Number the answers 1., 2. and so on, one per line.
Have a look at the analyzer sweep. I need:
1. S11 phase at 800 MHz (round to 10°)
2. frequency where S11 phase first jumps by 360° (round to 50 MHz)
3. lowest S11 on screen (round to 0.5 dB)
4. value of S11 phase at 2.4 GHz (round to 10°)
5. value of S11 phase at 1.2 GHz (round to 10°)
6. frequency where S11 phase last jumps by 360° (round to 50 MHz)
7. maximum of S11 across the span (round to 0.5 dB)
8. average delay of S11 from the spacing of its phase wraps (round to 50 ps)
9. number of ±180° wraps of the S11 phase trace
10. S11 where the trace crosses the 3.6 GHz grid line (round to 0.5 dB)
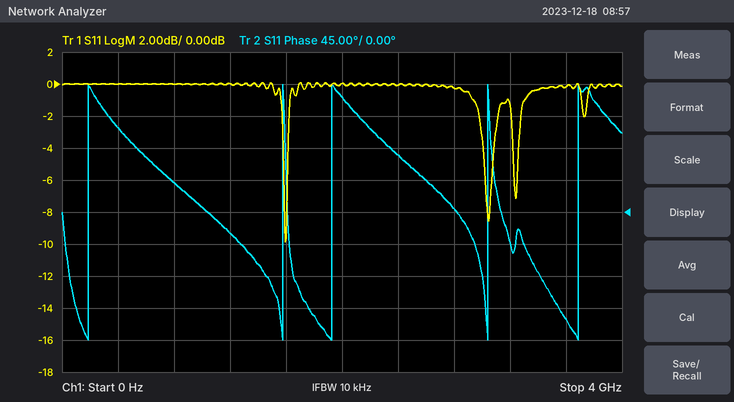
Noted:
1. 40°
2. 200 MHz
3. -10.0 dB
4. 80°
5. -30°
6. 3.70 GHz
7. 0.0 dB
8. 1.15 ns
9. 5
10. 0.0 dB
